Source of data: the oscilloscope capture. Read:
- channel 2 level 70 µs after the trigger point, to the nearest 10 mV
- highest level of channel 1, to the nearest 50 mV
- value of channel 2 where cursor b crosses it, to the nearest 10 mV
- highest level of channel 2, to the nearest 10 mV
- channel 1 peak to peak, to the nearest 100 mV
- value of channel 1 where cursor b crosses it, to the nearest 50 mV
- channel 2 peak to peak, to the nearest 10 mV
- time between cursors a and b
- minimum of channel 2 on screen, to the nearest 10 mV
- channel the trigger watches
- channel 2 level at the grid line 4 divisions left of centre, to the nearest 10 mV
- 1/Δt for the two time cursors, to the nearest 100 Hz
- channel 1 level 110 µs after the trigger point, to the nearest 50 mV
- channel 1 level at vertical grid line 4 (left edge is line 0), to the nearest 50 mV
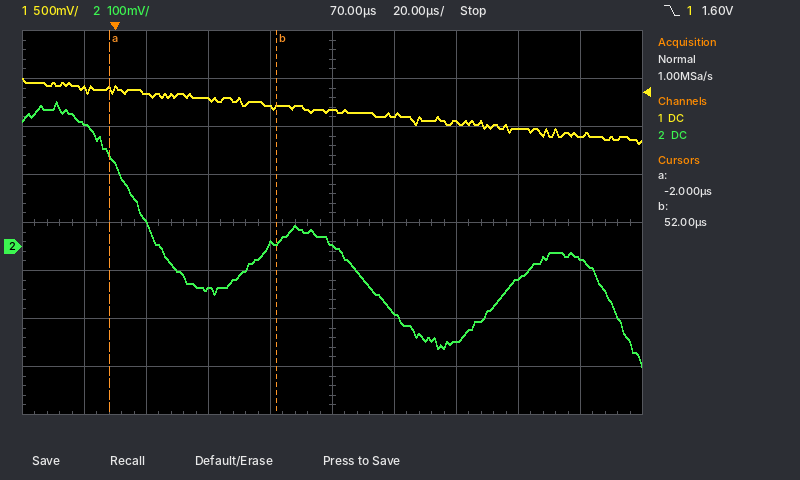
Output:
0 mV
1.75 V
10 mV
300 mV
700 mV
1.45 V
550 mV
54 µs
-250 mV
channel 1
260 mV
18.5 kHz
1.30 V
1.45 V
